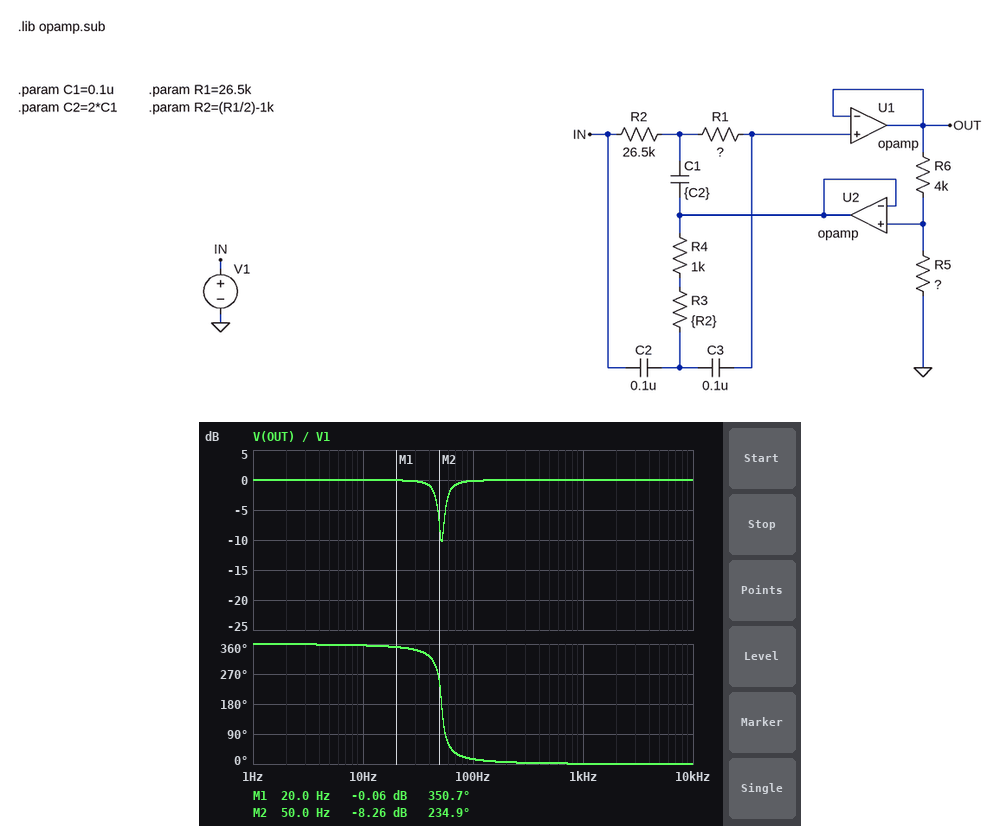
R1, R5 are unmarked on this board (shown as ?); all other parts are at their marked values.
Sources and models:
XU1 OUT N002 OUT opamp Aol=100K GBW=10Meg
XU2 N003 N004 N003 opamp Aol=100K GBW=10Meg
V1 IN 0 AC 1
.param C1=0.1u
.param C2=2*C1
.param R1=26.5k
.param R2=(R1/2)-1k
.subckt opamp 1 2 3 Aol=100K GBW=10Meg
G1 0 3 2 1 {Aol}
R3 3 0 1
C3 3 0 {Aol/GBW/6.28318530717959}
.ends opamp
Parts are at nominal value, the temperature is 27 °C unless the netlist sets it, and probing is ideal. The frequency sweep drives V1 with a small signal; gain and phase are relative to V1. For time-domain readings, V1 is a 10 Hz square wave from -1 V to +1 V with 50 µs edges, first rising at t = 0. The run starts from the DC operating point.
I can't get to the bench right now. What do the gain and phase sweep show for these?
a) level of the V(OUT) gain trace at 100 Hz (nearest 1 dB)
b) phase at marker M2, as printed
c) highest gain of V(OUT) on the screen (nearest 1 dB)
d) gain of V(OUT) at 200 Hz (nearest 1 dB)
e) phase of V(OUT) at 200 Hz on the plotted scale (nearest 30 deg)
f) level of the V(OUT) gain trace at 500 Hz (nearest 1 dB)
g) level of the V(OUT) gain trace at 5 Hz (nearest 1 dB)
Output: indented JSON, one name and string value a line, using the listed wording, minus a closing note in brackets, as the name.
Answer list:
{
  "level of the V(OUT) gain trace at 100 Hz": "0 dB",
  "phase at marker M2, as printed": "234.9 deg",
  "highest gain of V(OUT) on the screen": "0 dB",
  "gain of V(OUT) at 200 Hz": "0 dB",
  "phase of V(OUT) at 200 Hz on the plotted scale": "0 deg",
  "level of the V(OUT) gain trace at 500 Hz": "0 dB",
  "level of the V(OUT) gain trace at 5 Hz": "0 dB"
}
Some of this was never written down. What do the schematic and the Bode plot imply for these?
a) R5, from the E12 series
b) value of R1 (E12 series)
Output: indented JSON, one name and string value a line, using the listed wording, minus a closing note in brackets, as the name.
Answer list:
{
  "R5, from the E12 series": "39 kΩ",
  "value of R1": "39 kΩ"
}
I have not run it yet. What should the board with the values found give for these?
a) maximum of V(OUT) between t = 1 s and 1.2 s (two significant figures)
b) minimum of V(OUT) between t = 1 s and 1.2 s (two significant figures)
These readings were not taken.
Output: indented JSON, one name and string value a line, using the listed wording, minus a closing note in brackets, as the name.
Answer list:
{
  "maximum of V(OUT) between t = 1 s and 1.2 s": "1.4 V",
  "minimum of V(OUT) between t = 1 s and 1.2 s": "-1.4 V"
}
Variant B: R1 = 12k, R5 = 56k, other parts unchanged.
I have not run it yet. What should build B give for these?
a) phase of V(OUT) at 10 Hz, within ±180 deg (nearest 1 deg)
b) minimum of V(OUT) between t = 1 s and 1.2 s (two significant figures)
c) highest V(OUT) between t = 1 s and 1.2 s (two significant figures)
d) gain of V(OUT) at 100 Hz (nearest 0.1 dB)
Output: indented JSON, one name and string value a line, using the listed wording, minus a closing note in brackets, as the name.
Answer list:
{
  "phase of V(OUT) at 10 Hz, within ±180 deg": "-2 deg",
  "minimum of V(OUT) between t = 1 s and 1.2 s": "-1.2 V",
  "highest V(OUT) between t = 1 s and 1.2 s": "1.2 V",
  "gain of V(OUT) at 100 Hz": "-3.0 dB"
}
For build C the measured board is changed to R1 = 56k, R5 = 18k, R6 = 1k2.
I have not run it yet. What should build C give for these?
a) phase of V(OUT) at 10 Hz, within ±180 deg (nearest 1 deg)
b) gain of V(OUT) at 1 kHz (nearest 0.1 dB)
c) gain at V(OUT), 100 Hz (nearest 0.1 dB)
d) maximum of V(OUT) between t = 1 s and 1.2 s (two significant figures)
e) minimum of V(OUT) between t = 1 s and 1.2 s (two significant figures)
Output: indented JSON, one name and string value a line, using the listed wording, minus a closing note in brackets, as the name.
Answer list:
{
  "phase of V(OUT) at 10 Hz, within ±180 deg": "-3 deg",
  "gain of V(OUT) at 1 kHz": "0 dB",
  "gain at V(OUT), 100 Hz": "0 dB",
  "maximum of V(OUT) between t = 1 s and 1.2 s": "1.3 V",
  "minimum of V(OUT) between t = 1 s and 1.2 s": "-1.3 V"
}
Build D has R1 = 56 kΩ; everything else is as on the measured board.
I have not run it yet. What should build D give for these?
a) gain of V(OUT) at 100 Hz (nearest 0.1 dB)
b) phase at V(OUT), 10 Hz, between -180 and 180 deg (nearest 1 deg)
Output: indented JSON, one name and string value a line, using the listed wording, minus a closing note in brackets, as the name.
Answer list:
{
  "gain of V(OUT) at 100 Hz": "-0.1 dB",
  "phase at V(OUT), 10 Hz, between -180 and 180 deg": "-5 deg"
}
